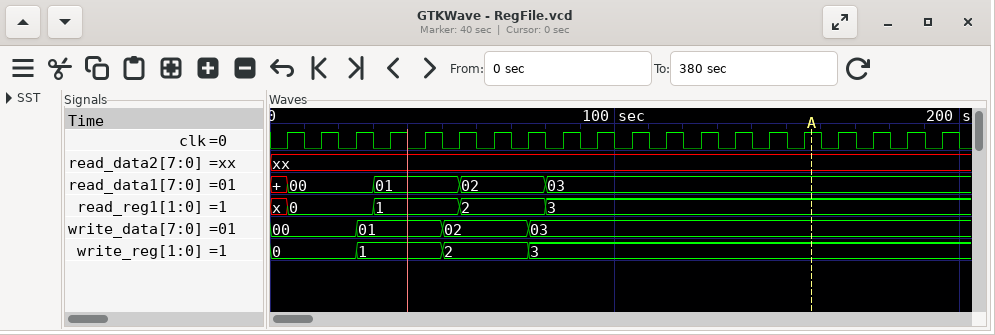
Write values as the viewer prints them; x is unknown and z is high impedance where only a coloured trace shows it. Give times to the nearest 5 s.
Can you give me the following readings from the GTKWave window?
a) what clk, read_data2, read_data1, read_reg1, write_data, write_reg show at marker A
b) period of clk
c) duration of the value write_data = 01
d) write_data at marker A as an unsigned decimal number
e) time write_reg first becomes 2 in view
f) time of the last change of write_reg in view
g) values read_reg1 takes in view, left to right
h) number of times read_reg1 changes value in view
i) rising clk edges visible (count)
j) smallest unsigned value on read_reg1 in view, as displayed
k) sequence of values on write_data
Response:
clk=1, read_data2=xx, read_data1=03, read_reg1=3, write_data=03, write_reg=3
10 s
25 s
3
50 s
75 s
x, 0, 1, 2, 3
4
20
0
00, 01, 02, 03
